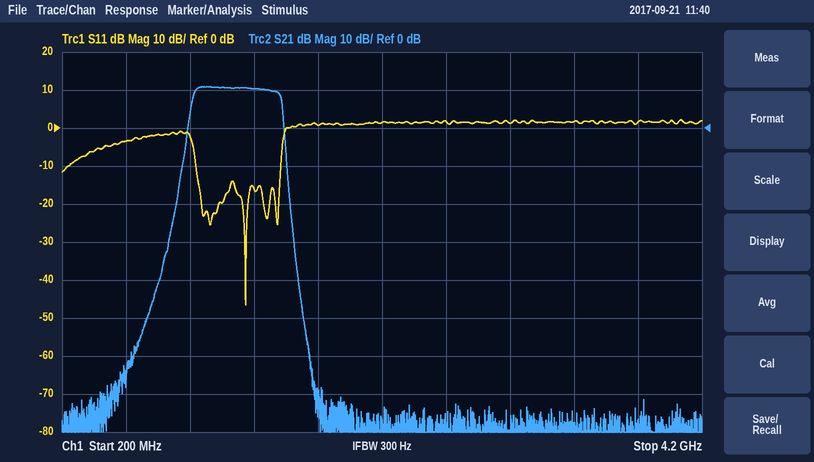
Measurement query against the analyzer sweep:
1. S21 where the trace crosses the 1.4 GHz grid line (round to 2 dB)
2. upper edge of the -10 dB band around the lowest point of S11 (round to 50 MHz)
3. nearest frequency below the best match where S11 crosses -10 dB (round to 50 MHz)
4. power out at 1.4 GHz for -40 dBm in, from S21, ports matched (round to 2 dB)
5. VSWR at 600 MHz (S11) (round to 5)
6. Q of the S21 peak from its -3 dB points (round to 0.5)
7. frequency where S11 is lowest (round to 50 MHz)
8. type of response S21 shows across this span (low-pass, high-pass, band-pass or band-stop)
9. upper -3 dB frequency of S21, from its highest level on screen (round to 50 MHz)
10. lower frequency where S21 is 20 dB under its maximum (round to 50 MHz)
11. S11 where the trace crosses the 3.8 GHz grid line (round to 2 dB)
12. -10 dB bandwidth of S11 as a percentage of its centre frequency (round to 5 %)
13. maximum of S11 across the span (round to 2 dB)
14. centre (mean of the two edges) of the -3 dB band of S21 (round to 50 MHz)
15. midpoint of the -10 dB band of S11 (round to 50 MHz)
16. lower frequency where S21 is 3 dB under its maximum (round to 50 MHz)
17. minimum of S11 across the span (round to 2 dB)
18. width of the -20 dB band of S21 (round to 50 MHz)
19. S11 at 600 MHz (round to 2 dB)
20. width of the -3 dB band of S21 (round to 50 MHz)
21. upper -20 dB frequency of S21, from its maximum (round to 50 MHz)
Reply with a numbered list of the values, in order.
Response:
1. 10 dB
2. 1.55 GHz
3. 1.05 GHz
4. -30 dBm
5. 5
6. 2.5
7. 1.35 GHz
8. band-pass
9. 1.55 GHz
10. 950 MHz
11. 2 dB
12. 40 %
13. 2 dB
14. 1.30 GHz
15. 1.30 GHz
16. 1.00 GHz
17. -46 dB
18. 650 MHz
19. -4 dB
20. 550 MHz
21. 1.60 GHz
